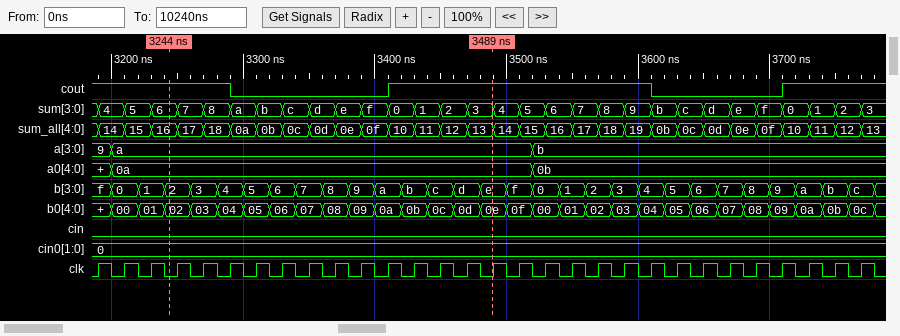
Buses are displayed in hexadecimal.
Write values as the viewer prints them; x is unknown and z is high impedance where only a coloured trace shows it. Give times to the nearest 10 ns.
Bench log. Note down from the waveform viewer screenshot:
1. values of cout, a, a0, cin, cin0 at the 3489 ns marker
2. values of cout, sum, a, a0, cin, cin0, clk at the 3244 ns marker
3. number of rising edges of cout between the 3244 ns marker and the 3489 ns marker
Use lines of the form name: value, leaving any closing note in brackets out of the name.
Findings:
values of cout, a, a0, cin, cin0 at the 3489 ns marker: cout=1, a=a, a0=0a, cin=0, cin0=0
values of cout, sum, a, a0, cin, cin0, clk at the 3244 ns marker: cout=1, sum=6, a=a, a0=0a, cin=0, cin0=0, clk=0
number of rising edges of cout between the 3244 ns marker and the 3489 ns marker: 1
